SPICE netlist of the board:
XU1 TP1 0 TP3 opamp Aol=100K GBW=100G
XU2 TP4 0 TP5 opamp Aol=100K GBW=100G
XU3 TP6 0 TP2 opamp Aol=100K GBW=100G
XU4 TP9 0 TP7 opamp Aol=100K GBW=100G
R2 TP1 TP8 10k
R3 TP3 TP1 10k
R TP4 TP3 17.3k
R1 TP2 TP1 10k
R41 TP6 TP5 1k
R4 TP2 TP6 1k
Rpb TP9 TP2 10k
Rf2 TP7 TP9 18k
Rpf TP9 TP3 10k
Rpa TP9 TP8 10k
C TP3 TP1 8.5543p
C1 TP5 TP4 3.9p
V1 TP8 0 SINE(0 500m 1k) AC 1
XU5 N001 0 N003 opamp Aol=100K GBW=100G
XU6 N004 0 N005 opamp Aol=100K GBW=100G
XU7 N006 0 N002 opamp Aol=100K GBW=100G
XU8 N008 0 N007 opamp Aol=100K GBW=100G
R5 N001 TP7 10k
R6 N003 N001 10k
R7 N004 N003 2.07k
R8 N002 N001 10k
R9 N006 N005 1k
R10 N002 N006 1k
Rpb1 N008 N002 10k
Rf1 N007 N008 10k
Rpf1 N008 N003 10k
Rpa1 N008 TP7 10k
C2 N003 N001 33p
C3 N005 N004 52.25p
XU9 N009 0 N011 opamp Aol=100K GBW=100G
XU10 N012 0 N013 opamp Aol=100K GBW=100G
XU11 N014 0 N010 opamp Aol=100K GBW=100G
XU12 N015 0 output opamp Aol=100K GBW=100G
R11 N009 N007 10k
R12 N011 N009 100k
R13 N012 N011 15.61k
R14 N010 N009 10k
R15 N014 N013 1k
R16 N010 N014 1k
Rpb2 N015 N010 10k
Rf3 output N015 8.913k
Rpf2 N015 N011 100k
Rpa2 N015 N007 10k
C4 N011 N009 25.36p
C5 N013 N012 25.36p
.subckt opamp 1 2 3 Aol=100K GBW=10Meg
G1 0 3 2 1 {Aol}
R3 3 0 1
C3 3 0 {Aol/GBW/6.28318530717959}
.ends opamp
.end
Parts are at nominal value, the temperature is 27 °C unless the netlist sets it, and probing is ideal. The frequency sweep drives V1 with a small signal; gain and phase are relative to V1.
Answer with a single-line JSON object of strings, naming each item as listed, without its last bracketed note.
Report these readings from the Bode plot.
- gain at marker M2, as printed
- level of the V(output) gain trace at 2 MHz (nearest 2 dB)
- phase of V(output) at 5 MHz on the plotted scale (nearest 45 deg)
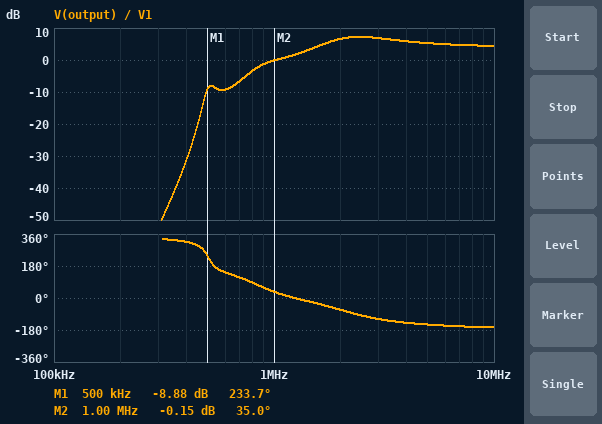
{"gain at marker M2, as printed": "-0.15 dB", "level of the V(output) gain trace at 2 MHz": "6 dB", "phase of V(output) at 5 MHz on the plotted scale": "-135 deg"}
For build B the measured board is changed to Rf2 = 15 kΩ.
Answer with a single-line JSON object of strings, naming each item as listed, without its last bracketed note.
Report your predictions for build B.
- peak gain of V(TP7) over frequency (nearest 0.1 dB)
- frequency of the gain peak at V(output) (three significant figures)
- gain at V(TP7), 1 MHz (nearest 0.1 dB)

{"peak gain of V(TP7) over frequency": "5.5 dB", "frequency of the gain peak at V(output)": "2.44 MHz", "gain at V(TP7), 1 MHz": "-8.2 dB"}
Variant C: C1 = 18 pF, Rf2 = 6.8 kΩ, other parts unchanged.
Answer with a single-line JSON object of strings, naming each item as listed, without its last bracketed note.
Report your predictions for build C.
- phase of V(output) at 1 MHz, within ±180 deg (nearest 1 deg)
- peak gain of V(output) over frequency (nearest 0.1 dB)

{"phase of V(output) at 1 MHz, within ±180 deg": "-28 deg", "peak gain of V(output) over frequency": "-2.2 dB"}
